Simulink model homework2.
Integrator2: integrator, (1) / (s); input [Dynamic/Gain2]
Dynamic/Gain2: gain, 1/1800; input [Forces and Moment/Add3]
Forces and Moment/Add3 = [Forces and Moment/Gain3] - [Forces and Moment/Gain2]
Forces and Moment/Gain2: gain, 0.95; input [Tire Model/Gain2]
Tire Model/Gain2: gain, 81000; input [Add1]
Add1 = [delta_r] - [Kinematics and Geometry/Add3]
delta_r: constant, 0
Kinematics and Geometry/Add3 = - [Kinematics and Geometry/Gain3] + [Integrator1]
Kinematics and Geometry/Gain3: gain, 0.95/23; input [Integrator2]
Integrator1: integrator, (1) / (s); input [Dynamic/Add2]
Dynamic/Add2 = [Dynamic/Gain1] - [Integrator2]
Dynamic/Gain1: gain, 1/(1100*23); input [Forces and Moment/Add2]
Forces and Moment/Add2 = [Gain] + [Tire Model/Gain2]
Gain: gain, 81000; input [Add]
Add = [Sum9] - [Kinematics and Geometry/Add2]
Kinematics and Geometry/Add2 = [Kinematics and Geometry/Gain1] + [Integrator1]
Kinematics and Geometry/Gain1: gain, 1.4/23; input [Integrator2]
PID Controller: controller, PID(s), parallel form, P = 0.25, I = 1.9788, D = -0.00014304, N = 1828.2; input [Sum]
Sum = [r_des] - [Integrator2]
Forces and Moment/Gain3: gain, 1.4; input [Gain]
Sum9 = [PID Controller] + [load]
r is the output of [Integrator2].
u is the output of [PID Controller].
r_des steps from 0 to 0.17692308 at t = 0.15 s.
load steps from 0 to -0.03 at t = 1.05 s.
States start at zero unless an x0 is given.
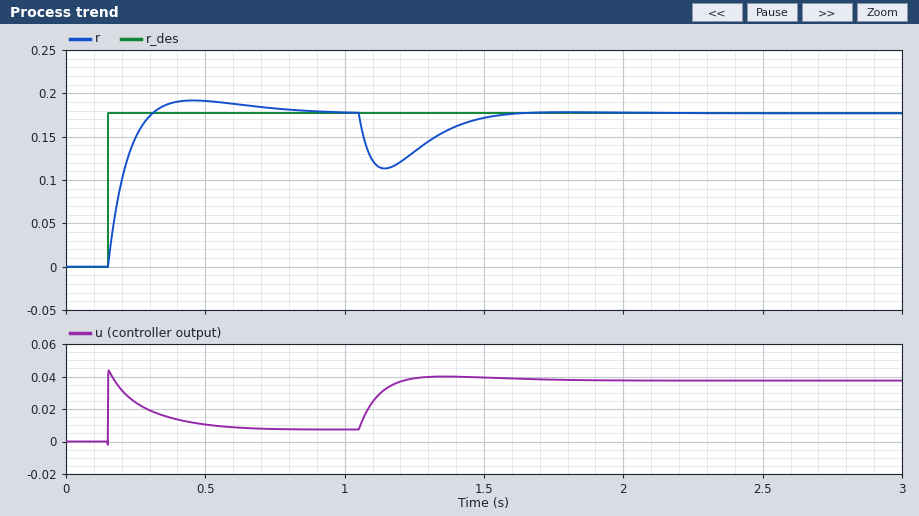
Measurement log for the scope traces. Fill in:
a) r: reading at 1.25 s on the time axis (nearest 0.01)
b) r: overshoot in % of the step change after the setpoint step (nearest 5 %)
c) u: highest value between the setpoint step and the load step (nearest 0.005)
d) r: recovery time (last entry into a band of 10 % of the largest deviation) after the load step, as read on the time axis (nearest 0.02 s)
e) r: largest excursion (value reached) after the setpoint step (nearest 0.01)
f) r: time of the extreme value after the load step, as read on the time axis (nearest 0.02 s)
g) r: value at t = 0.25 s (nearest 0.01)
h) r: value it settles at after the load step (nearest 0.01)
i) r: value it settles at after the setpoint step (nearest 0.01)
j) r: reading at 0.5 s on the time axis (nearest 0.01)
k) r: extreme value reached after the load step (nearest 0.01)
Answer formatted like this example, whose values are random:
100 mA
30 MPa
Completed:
0.13
10 %
0.045
1.48 s
0.19
1.14 s
0.15
0.18
0.18
0.19
0.11
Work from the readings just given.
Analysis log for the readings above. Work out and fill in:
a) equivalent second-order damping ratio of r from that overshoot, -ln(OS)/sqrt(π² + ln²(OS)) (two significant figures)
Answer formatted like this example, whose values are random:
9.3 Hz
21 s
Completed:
0.59
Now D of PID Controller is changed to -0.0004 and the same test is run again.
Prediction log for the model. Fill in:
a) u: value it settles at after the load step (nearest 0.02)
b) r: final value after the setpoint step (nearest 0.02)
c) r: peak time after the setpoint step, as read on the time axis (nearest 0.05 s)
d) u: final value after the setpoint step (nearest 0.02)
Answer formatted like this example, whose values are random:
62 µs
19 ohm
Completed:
0.04
0.18
0.45 s
0.00
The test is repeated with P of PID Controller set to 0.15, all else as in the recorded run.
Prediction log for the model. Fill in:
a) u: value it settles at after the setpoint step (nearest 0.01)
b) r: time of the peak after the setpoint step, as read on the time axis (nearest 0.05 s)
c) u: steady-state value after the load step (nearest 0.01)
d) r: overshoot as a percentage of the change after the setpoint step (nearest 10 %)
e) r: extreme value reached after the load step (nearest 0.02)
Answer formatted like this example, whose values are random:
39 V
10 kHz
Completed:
0.01
0.45 s
0.04
20 %
0.10
